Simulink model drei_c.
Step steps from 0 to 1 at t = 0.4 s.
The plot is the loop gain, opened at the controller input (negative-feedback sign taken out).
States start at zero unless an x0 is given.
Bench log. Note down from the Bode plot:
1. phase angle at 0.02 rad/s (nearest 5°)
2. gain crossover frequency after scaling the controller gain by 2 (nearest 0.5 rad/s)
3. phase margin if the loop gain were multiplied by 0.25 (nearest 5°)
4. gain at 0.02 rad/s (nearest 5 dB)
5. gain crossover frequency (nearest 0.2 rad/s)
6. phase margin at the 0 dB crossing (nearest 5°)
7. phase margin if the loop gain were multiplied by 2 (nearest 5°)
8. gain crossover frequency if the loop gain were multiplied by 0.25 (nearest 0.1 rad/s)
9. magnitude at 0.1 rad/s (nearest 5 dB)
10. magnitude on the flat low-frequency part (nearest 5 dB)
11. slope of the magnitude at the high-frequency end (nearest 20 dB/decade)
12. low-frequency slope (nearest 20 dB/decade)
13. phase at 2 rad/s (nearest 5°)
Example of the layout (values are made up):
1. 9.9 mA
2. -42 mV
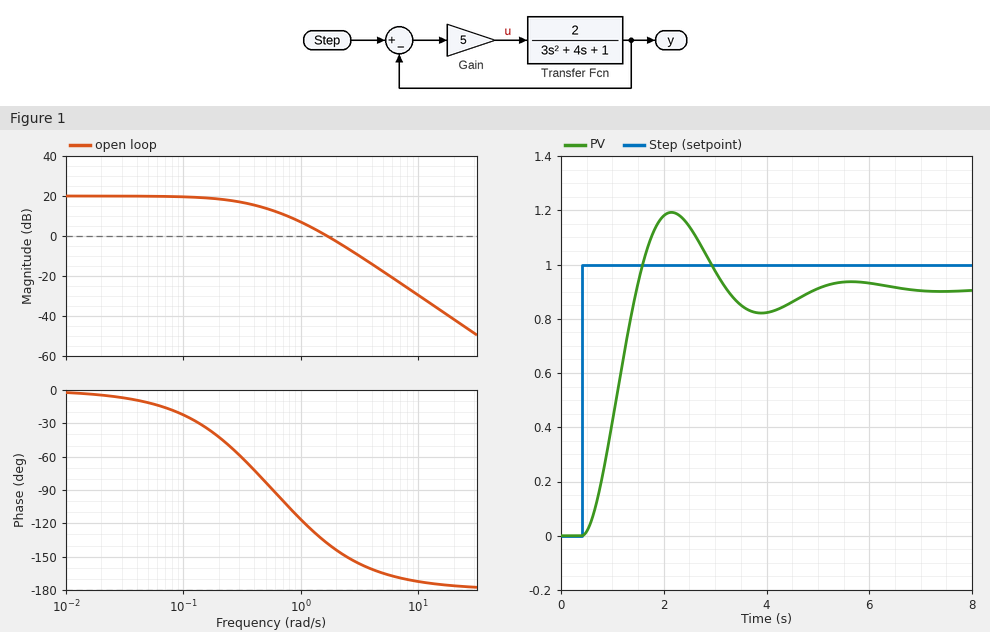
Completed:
1. -5°
2. 2.5 rad/s
3. 85°
4. 20 dB
5. 1.6 rad/s
6. 40°
7. 30°
8. 0.6 rad/s
9. 20 dB
10. 20 dB
11. -40 dB/decade
12. 0 dB/decade
13. -145°
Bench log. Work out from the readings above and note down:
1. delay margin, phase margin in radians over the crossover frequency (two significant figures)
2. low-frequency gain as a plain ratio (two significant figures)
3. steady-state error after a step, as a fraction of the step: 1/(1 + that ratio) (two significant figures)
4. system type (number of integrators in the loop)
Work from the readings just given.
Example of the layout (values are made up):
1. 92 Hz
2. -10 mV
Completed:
1. 0.44 s
2. 10
3. 0.091
4. 0
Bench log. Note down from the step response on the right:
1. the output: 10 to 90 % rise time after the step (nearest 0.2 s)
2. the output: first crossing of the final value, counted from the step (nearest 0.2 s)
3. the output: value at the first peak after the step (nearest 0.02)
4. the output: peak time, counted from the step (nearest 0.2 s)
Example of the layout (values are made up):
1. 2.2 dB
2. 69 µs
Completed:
1. 0.8 s
2. 1.0 s
3. 1.20
4. 1.8 s
